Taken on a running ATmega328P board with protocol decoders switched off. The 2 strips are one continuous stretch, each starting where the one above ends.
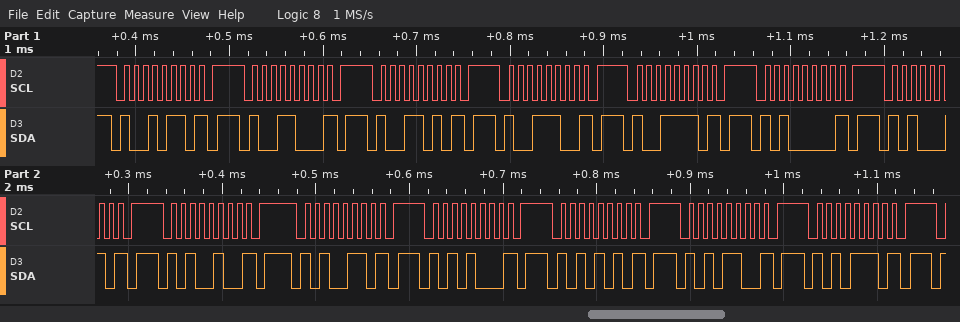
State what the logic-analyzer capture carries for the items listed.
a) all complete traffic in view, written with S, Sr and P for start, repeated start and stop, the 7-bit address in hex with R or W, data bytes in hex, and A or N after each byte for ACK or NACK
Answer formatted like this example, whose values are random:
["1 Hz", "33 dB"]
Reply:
["S 4BW N P S 4CW N P S 4DW N P S 4EW N P S 4FW N P S 50W N P S 51W N P S 52W N P S 53W N P S 54W N P S 55W N P S 56W N P S 57W N P"]
